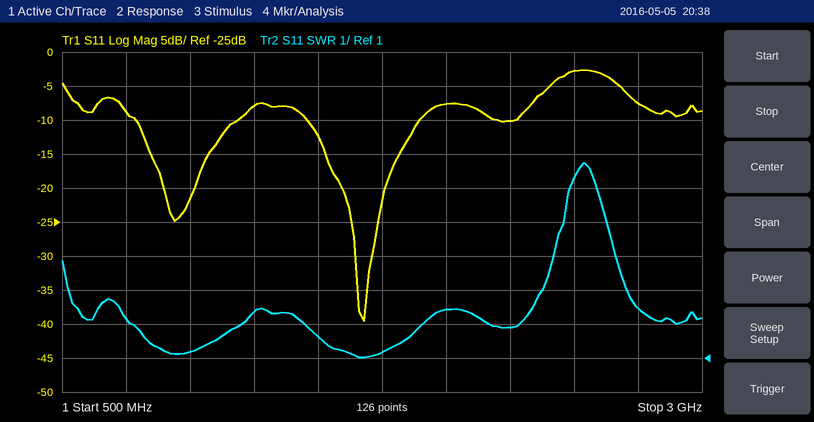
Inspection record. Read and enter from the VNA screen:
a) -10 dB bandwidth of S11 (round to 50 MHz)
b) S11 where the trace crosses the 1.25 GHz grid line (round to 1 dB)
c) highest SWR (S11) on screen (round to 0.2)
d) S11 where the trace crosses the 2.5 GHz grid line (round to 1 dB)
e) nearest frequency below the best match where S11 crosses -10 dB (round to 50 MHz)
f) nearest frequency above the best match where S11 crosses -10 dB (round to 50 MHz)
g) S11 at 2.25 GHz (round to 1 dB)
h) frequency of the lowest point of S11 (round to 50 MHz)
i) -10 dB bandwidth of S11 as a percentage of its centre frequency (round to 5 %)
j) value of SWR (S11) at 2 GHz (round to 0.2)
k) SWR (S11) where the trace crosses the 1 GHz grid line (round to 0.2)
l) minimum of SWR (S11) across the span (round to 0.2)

450 MHz
-8 dB
6.8
-3 dB
1.45 GHz
1.90 GHz
-10 dB
1.70 GHz
25 %
2.4
1.2
1.0
